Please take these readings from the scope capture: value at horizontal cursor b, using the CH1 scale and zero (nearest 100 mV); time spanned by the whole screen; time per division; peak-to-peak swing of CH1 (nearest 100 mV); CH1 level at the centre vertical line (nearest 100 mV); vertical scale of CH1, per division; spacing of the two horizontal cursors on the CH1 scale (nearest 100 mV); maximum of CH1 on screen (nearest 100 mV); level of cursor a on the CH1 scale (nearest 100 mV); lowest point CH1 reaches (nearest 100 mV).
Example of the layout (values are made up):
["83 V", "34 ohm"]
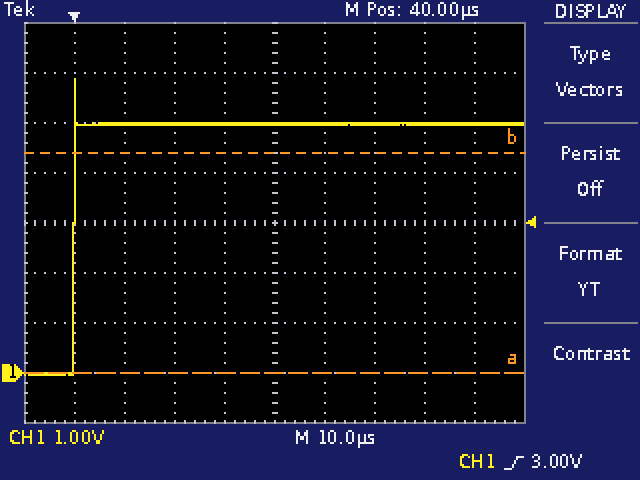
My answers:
["4.4 V", "100 µs", "10 µs", "5.9 V", "5.0 V", "1 V", "4.4 V", "5.9 V", "0.0 V", "0.0 V"]
